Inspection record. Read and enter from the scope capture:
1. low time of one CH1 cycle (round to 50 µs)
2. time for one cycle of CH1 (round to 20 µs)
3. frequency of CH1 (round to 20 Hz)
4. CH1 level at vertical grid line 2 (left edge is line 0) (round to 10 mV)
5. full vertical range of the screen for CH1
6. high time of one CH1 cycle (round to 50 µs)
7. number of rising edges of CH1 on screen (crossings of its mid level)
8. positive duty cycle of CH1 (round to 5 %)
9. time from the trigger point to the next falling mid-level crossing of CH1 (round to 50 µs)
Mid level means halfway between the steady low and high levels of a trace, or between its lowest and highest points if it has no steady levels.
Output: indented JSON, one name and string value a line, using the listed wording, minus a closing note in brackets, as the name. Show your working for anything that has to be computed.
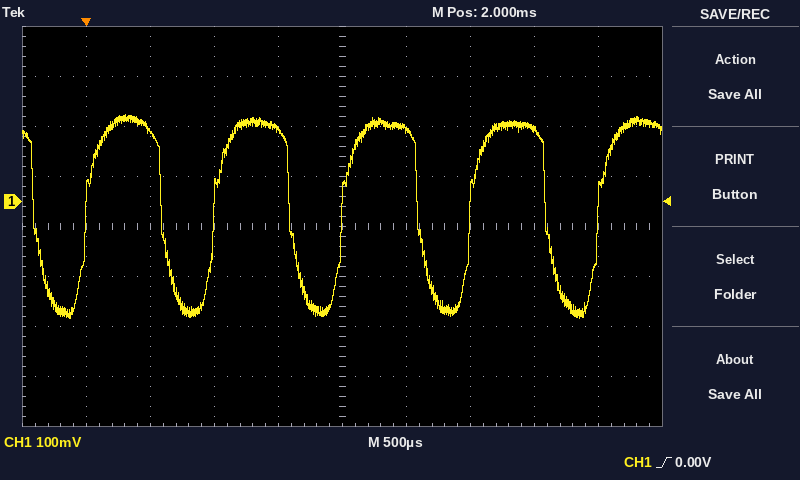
{
  "low time of one CH1 cycle": "400 µs",
  "time for one cycle of CH1": "1.00 ms",
  "frequency of CH1": "1 / 1.00 ms ≈ 1.00 kHz",
  "CH1 level at vertical grid line 2 (left edge is line 0)": "140 mV",
  "full vertical range of the screen for CH1": "800 mV",
  "high time of one CH1 cycle": "600 µs",
  "number of rising edges of CH1 on screen": "5",
  "positive duty cycle of CH1": "600 µs / 1.00 ms ≈ 60 %",
  "time from the trigger point to the next falling mid-level crossing of CH1": "600 µs"
}
